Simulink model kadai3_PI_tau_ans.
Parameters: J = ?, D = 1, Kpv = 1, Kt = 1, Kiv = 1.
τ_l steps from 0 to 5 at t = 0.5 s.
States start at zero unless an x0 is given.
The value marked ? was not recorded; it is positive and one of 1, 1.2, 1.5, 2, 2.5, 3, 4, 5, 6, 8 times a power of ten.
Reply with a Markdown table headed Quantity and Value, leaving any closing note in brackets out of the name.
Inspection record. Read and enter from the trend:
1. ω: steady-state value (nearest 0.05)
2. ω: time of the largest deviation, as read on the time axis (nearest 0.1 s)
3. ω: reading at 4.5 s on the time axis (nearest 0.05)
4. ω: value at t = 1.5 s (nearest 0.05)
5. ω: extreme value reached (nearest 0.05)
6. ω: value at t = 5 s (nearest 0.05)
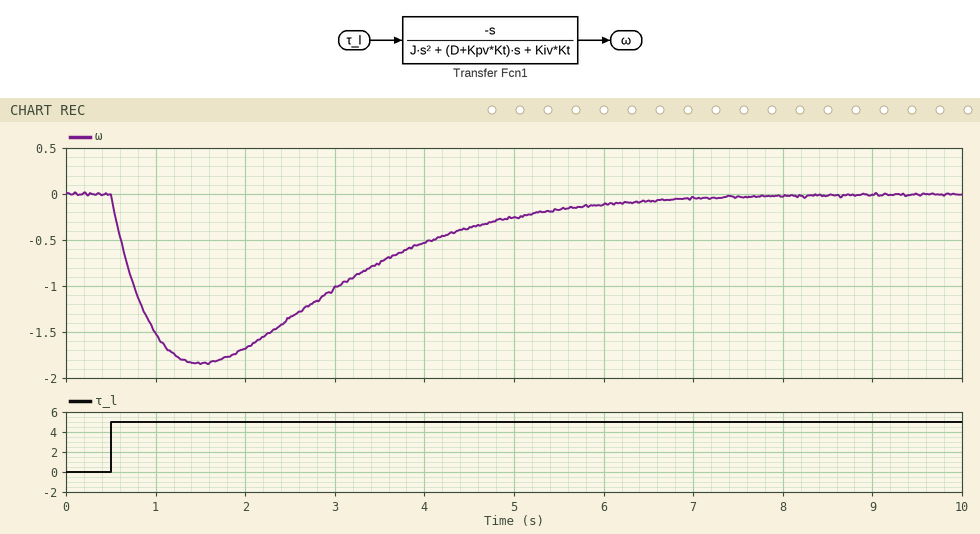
| Quantity | Value |
|---|---|
| ω: steady-state value | 0.00 |
| ω: time of the largest deviation, as read on the time axis | 1.5 s |
| ω: reading at 4.5 s on the time axis | -0.35 |
| ω: value at t = 1.5 s | -1.85 |
| ω: extreme value reached | -1.85 |
| ω: value at t = 5 s | -0.25 |
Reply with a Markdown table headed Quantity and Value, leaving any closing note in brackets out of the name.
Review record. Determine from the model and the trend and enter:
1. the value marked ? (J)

| Quantity | Value |
|---|---|
| the value marked ? | 1 |
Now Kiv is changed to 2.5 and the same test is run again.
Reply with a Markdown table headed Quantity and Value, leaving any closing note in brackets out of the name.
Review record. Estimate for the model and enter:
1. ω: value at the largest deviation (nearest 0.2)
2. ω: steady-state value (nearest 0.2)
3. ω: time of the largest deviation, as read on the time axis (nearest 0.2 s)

| Quantity | Value |
|---|---|
| ω: value at the largest deviation | -1.6 |
| ω: steady-state value | 0.0 |
| ω: time of the largest deviation, as read on the time axis | 1.2 s |
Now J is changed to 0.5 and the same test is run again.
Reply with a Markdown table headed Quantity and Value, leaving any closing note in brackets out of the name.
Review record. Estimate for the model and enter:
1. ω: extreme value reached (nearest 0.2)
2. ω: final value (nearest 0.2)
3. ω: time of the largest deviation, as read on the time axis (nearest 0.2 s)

| Quantity | Value |
|---|---|
| ω: extreme value reached | -2.0 |
| ω: final value | 0.0 |
| ω: time of the largest deviation, as read on the time axis | 1.2 s |
